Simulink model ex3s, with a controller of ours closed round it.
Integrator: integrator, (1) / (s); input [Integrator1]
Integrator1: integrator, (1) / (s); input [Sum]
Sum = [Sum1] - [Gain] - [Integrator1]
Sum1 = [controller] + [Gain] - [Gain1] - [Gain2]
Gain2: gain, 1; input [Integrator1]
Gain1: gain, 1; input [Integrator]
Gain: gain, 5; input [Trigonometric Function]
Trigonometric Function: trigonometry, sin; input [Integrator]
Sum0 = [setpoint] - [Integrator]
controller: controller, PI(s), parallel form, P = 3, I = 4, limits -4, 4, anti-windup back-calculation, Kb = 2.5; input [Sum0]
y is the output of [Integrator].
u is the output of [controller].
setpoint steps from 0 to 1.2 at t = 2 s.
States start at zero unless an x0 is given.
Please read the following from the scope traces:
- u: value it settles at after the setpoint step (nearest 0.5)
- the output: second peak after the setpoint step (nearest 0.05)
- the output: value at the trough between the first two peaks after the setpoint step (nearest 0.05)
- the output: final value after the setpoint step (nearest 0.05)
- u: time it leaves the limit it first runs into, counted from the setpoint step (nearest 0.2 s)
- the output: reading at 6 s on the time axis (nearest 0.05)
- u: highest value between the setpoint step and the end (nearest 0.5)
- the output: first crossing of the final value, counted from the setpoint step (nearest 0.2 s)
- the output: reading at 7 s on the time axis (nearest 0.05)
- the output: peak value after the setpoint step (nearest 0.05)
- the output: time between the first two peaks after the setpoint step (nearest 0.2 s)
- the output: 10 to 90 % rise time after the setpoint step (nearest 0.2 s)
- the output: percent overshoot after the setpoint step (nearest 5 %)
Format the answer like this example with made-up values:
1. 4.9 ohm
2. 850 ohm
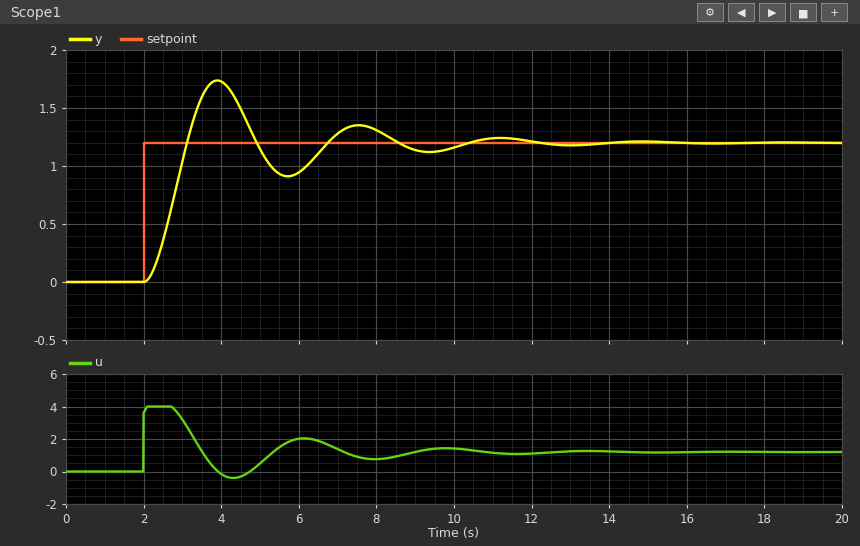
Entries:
1. 1.0
2. 1.35
3. 0.90
4. 1.20
5. 0.8 s
6. 0.95
7. 4.0
8. 1.2 s
9. 1.30
10. 1.75
11. 3.6 s
12. 0.8 s
13. 45 %
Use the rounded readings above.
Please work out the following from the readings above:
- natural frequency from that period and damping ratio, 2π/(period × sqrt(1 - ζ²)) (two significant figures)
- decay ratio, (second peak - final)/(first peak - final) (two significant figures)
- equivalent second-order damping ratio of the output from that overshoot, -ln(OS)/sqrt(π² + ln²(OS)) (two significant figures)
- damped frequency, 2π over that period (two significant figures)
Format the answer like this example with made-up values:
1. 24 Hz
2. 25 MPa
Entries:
1. 1.8 rad/s
2. 0.27
3. 0.25
4. 1.7 rad/s
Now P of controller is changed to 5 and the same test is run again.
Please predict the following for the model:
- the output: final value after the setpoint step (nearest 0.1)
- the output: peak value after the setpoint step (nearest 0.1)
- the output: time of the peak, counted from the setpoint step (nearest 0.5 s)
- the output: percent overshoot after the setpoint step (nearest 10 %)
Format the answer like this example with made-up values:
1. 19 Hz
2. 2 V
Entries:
1. 1.2
2. 1.4
3. 1.5 s
4. 20 %
